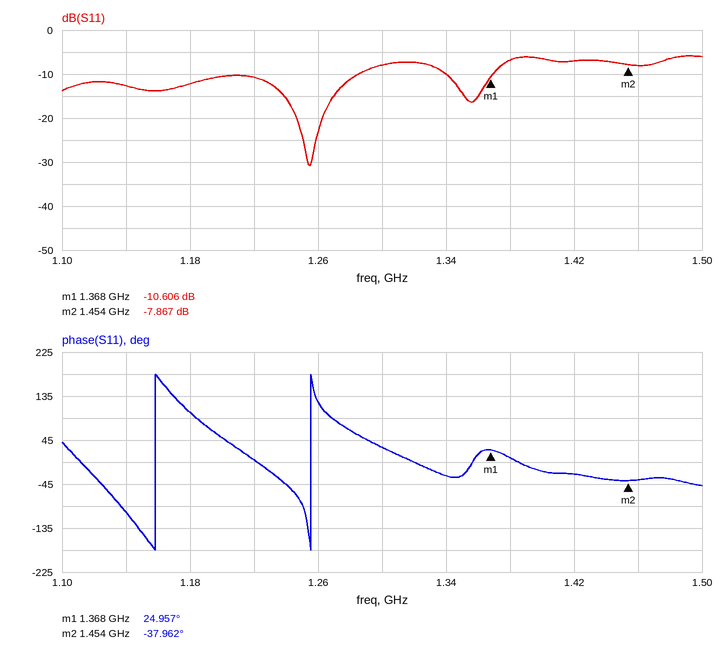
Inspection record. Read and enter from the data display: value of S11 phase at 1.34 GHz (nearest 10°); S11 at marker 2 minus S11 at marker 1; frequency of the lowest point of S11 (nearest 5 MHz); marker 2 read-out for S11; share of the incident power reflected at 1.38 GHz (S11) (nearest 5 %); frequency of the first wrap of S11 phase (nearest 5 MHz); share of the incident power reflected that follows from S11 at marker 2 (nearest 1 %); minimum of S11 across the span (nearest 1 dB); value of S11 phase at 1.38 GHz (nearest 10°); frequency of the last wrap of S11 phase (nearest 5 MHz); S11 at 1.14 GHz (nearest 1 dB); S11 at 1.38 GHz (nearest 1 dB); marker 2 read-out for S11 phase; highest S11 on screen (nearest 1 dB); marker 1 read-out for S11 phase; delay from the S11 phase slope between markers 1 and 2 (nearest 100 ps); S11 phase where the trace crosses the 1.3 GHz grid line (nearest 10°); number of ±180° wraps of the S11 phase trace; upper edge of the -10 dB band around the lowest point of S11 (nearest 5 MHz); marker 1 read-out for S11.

-30°
2.739 dB
1.255 GHz
-7.867 dB
20 %
1.160 GHz
16 %
-31 dB
10°
1.255 GHz
-13 dB
-7 dB
-37.962°
-6 dB
24.957°
2.0 ns
30°
2
1.285 GHz
-10.606 dB
